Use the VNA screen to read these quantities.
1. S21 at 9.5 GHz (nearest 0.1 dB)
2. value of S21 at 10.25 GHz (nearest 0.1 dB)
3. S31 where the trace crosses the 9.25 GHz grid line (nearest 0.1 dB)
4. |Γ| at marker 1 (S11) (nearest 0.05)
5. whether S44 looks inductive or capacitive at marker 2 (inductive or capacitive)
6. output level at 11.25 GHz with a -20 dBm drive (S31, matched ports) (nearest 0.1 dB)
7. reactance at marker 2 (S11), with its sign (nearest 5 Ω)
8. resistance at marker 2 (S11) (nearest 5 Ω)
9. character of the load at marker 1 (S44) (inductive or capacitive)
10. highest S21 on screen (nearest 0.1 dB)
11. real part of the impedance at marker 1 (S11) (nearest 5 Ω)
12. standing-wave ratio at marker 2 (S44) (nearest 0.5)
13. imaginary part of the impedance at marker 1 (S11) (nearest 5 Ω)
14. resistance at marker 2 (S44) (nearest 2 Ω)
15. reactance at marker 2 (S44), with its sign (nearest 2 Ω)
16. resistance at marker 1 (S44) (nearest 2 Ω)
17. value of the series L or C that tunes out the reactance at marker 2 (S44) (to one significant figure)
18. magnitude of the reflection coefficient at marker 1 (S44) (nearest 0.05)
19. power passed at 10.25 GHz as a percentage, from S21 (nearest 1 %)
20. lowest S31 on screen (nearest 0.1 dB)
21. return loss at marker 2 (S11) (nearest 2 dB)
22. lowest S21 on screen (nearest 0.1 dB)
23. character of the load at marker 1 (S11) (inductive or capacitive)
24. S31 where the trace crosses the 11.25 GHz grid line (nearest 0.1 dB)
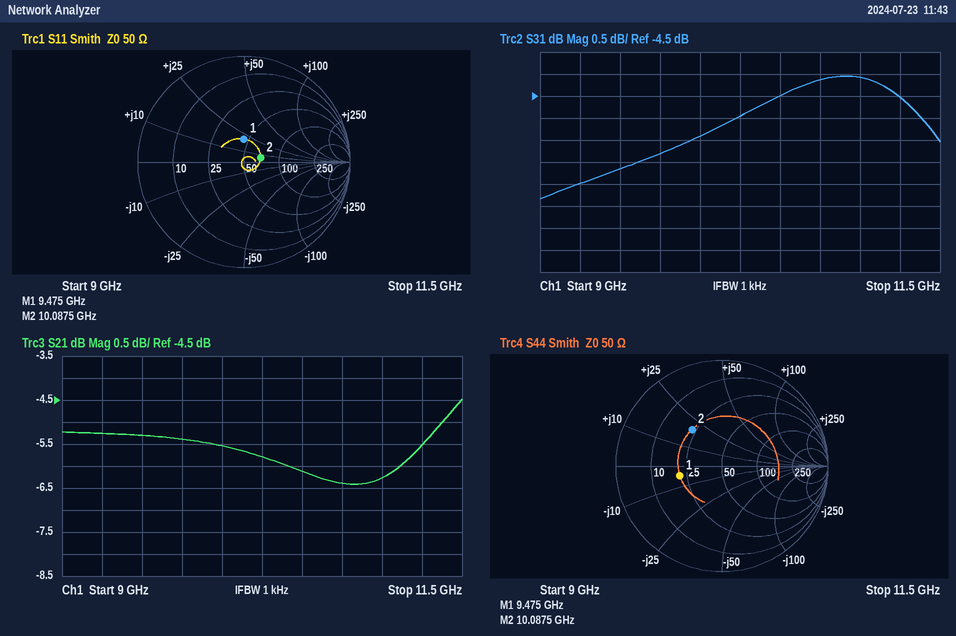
-5.3 dB
-5.8 dB
-6.5 dB
0.20
inductive
-24.5 dBm
+5 Ω
70 Ω
capacitive
-4.5 dB
45 Ω
2.5
+20 Ω
22 Ω
+20 Ω
22 Ω
800 fF
0.40
26 %
-6.8 dB
16 dB
-6.4 dB
inductive
-4.5 dB
